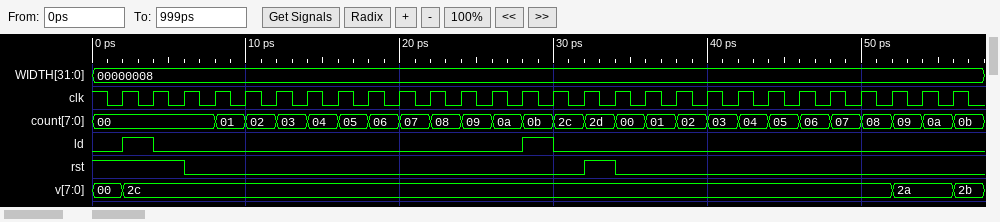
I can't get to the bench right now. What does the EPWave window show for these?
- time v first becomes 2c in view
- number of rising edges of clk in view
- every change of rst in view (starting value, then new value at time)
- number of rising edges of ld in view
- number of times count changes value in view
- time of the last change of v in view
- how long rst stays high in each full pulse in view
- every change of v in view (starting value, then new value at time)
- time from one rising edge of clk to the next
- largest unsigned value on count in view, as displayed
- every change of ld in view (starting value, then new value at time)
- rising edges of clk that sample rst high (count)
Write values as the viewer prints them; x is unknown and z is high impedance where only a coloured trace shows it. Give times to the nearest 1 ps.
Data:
2 ps
28
1, 0 at 6 ps, 1 at 32 ps, 0 at 34 ps
2
25
56 ps
2 ps
00, 2c at 2 ps, 2a at 52 ps, 2b at 56 ps
2 ps
2d
0, 1 at 2 ps, 0 at 4 ps, 1 at 28 ps, 0 at 30 ps
4
